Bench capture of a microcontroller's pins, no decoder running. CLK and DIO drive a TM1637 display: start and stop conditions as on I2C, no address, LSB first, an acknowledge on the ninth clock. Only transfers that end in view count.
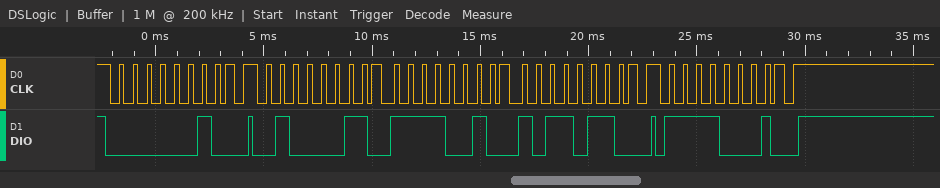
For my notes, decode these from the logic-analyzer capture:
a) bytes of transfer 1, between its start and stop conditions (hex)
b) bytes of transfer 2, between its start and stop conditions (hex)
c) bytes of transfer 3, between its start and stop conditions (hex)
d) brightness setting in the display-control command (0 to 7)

40
C2 4F 6D
8F
7
